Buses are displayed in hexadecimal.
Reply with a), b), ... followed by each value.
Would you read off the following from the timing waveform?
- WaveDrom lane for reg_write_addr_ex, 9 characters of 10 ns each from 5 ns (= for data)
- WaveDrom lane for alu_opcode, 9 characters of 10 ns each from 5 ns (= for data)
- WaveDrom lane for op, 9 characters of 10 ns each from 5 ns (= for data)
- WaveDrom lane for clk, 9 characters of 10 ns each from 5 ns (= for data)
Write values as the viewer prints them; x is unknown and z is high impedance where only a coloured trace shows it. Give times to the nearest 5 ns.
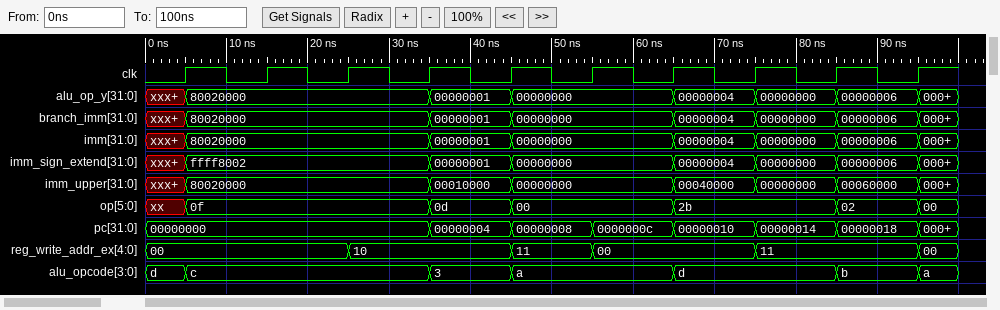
a) {name: 'reg_write_addr_ex', wave: '=.=.==.=.', data: '00 10 11 00 11'}
b) {name: 'alu_opcode', wave: '=..==.=.=', data: 'c 3 a d b'}
c) {name: 'op', wave: '=..==.=.=', data: '0f 0d 00 2b 02'}
d) {name: 'clk', wave: 'p........'}
